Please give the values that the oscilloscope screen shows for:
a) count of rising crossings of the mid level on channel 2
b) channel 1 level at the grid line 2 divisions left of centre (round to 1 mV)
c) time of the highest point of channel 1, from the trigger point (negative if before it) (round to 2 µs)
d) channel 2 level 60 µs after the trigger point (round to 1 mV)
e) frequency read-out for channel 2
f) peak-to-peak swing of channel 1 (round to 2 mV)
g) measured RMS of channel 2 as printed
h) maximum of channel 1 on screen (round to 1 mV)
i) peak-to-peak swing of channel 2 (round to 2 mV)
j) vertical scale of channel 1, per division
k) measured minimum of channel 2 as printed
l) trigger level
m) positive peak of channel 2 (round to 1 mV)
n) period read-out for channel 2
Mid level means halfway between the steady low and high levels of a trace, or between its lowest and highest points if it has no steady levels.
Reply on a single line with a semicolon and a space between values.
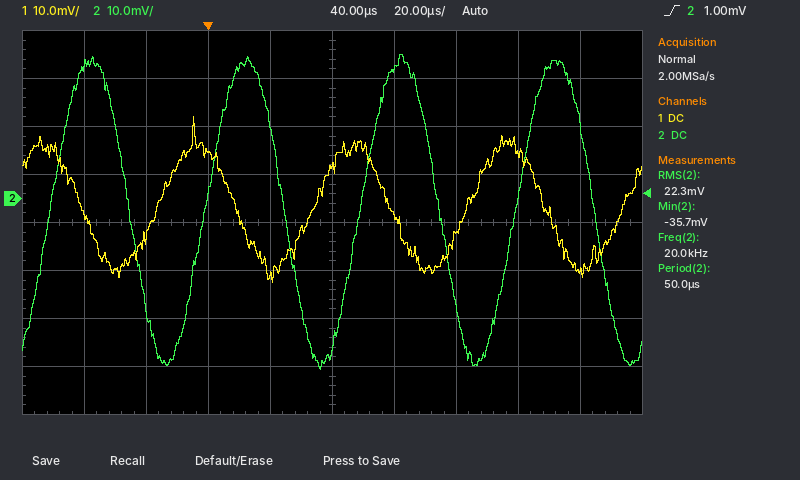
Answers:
4; 10 mV; -4 µs; 27 mV; 20.0 kHz; 34 mV; 22.3 mV; 17 mV; 66 mV; 10 mV; -35.7 mV; 1.00 mV; 30 mV; 50.0 µs
